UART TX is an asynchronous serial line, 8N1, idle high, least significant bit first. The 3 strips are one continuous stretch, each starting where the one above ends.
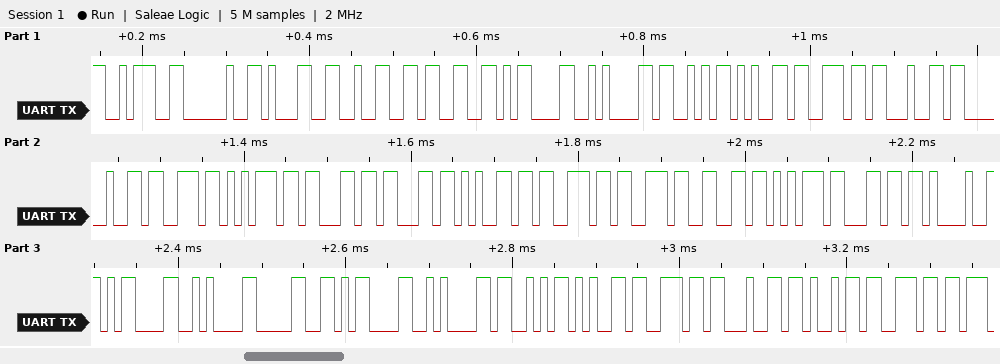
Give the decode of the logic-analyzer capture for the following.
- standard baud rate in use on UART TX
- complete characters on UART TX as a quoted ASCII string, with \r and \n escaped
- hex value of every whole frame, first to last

115200 baud
": 123\r\nSend successful!\r\n0\r\nSendin"
3A 20 31 32 33 0D 0A 53 65 6E 64 20 73 75 63 63 65 73 73 66 75 6C 21 0D 0A 30 0D 0A 53 65 6E 64 69 6E
